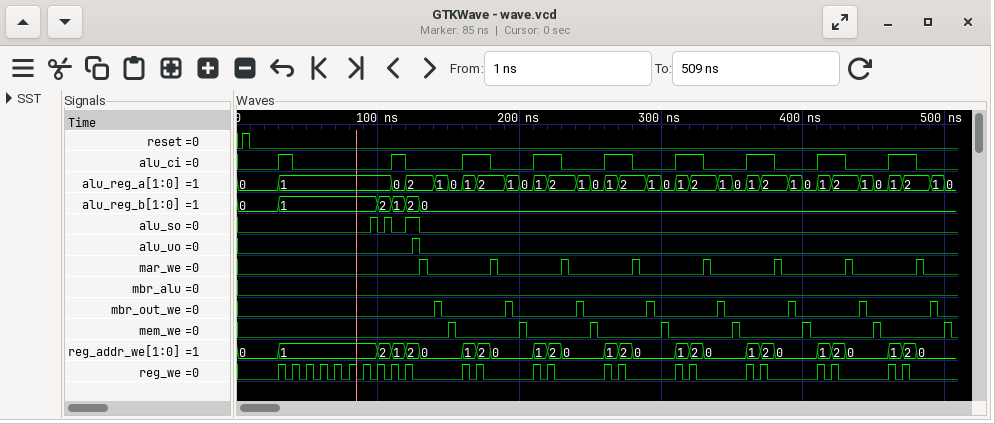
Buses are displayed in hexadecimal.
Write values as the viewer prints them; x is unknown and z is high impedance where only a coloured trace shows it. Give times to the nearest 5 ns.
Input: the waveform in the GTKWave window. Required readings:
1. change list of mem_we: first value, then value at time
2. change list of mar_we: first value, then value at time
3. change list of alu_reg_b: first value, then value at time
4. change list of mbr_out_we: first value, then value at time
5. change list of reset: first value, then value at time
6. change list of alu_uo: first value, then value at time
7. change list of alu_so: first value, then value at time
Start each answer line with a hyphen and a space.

- 0, 1 at 150 ns, 0 at 155 ns, 1 at 200 ns, 0 at 205 ns, 1 at 250 ns, 0 at 255 ns, 1 at 300 ns, 0 at 305 ns, 1 at 350 ns, 0 at 355 ns, 1 at 400 ns, 0 at 405 ns, 1 at 450 ns, 0 at 455 ns, 1 at 500 ns, 0 at 505 ns
- 0, 1 at 130 ns, 0 at 135 ns, 1 at 180 ns, 0 at 185 ns, 1 at 230 ns, 0 at 235 ns, 1 at 280 ns, 0 at 285 ns, 1 at 330 ns, 0 at 335 ns, 1 at 380 ns, 0 at 385 ns, 1 at 430 ns, 0 at 435 ns, 1 at 480 ns, 0 at 485 ns
- 0, 1 at 30 ns, 2 at 100 ns, 1 at 110 ns, 2 at 120 ns, 0 at 130 ns
- 0, 1 at 140 ns, 0 at 145 ns, 1 at 190 ns, 0 at 195 ns, 1 at 240 ns, 0 at 245 ns, 1 at 290 ns, 0 at 295 ns, 1 at 340 ns, 0 at 345 ns, 1 at 390 ns, 0 at 395 ns, 1 at 440 ns, 0 at 445 ns, 1 at 490 ns, 0 at 495 ns
- 0, 1 at 5 ns, 0 at 10 ns
- 0, 1 at 125 ns, 0 at 130 ns
- 0, 1 at 95 ns, 0 at 100 ns, 1 at 105 ns, 0 at 110 ns, 1 at 120 ns, 0 at 130 ns
